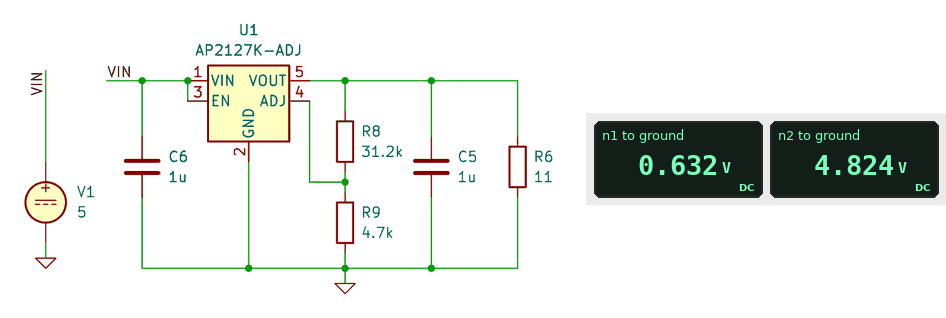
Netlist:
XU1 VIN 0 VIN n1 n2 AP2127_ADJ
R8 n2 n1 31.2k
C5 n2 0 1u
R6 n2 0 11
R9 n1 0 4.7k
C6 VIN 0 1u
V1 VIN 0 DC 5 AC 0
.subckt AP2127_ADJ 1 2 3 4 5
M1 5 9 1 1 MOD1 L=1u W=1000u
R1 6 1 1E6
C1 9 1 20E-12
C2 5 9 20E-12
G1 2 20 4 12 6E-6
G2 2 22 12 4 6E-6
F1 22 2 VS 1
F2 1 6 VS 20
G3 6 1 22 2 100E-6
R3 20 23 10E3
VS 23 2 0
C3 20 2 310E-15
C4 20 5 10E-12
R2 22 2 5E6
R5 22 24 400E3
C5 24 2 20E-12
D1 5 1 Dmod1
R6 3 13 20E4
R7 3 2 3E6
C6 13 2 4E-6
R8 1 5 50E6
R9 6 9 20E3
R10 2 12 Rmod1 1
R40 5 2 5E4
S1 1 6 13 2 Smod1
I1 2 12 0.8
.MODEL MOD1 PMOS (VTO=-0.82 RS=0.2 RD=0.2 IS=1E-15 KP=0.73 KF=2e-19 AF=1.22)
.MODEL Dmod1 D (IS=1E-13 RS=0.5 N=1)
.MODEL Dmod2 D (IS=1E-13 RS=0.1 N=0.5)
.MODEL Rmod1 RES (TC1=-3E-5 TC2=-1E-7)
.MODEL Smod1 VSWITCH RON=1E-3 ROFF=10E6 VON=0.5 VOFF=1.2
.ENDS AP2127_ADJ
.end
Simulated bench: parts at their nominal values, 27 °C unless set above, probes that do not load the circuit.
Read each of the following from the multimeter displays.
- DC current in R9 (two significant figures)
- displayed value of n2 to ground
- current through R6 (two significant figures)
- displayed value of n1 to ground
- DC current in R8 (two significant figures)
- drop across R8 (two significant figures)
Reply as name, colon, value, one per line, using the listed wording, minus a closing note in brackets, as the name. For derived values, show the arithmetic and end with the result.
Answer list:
DC current in R9: (632 mV) / 4.7 kΩ = 130 µA
displayed value of n2 to ground: 4.824 V
current through R6: (4.824 V) / 11 Ω = 440 mA
displayed value of n1 to ground: 0.632 V
DC current in R8: (4.824 V - 632 mV) / 31.2 kΩ = 130 µA
drop across R8: 4.824 V - 632 mV = 4.2 V
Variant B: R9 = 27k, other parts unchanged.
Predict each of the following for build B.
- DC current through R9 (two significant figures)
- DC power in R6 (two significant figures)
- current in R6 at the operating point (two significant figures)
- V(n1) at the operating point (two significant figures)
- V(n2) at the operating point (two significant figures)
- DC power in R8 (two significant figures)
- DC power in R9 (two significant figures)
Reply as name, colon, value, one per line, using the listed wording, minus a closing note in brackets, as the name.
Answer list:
DC current through R9: 30 µA
DC power in R6: 270 mW
current in R6 at the operating point: 160 mA
V(n1) at the operating point: 800 mV
V(n2) at the operating point: 1.7 V
DC power in R8: 27 µW
DC power in R9: 24 µW
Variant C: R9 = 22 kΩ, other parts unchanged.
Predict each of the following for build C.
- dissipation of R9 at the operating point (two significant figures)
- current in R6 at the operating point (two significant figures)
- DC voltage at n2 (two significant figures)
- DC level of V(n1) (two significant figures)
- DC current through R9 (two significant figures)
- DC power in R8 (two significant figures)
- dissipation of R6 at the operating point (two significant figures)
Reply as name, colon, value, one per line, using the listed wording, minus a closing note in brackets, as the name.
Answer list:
dissipation of R9 at the operating point: 29 µW
current in R6 at the operating point: 180 mA
DC voltage at n2: 1.9 V
DC level of V(n1): 800 mV
DC current through R9: 36 µA
DC power in R8: 41 µW
dissipation of R6 at the operating point: 340 mW
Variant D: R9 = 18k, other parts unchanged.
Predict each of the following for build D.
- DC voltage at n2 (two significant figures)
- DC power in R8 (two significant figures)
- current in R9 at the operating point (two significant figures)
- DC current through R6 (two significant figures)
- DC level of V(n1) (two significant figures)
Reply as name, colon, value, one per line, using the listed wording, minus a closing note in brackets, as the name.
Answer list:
DC voltage at n2: 2.2 V
DC power in R8: 62 µW
current in R9 at the operating point: 44 µA
DC current through R6: 200 mA
DC level of V(n1): 800 mV
